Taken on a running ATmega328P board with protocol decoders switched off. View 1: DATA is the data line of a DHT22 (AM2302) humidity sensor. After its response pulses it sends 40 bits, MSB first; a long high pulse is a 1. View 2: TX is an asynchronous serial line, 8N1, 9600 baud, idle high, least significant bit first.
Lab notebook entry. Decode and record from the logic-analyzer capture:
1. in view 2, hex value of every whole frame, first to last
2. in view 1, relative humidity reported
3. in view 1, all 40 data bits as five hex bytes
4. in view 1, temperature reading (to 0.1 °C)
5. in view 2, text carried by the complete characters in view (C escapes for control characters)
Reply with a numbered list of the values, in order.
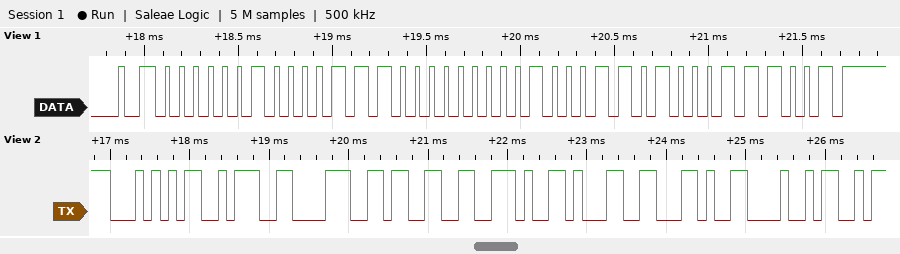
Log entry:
1. 54 3A 38 33 2E 31 2C 48
2. 54.0 %
3. 02 1C 01 1A 39
4. 28.2 °C
5. "T:83.1,H"
